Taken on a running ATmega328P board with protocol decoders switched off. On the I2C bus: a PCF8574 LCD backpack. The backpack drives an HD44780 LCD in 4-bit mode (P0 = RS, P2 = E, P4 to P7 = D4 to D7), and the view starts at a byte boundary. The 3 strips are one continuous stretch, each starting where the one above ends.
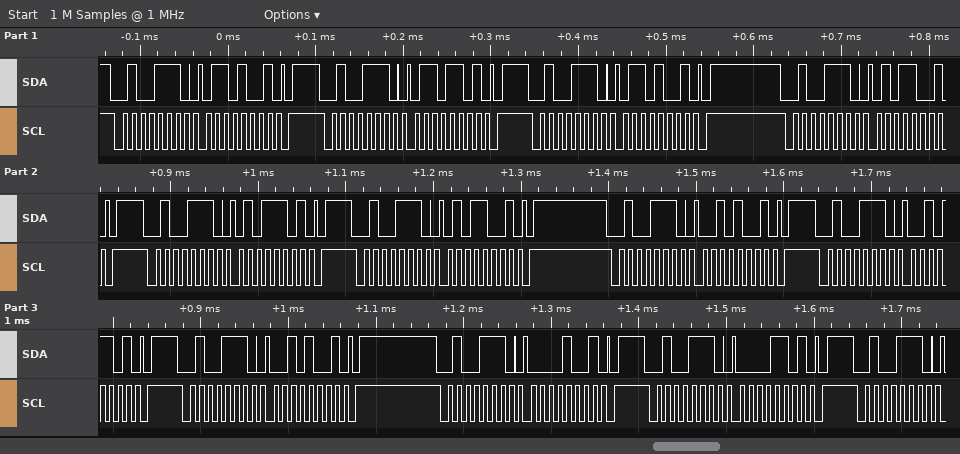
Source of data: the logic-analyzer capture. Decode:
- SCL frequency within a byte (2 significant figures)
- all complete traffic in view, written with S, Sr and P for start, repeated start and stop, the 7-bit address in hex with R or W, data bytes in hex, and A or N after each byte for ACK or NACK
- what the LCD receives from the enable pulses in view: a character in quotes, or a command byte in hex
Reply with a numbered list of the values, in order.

1. 100 kHz
2. S 27W A 69 A P S 27W A 6D A P S 27W A 69 A P S 27W A 59 A P S 27W A 5D A P S 27W A 59 A P S 27W A 29 A P S 27W A 2D A P S 27W A 29 A P S 27W A 09 A P S 27W A 0D A P S 27W A
3. 'e'
